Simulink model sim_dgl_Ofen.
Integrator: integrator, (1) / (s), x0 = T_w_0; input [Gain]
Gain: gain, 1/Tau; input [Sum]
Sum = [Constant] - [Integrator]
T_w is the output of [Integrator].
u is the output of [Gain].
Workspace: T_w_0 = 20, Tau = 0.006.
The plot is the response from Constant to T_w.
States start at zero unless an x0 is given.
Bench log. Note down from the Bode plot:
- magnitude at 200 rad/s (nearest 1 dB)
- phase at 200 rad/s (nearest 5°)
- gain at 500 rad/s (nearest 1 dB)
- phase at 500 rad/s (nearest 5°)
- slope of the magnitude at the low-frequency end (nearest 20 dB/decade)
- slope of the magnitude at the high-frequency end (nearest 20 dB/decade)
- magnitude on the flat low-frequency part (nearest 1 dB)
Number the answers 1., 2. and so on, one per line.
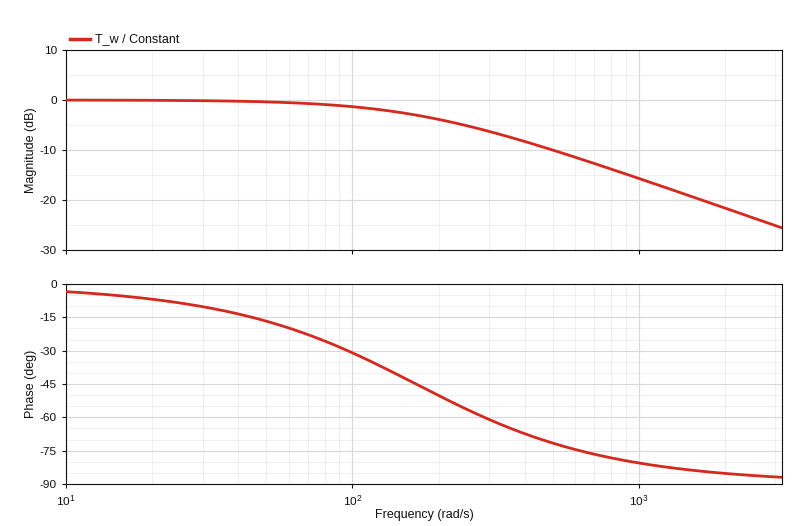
1. -4 dB
2. -50°
3. -10 dB
4. -70°
5. 0 dB/decade
6. -20 dB/decade
7. 0 dB
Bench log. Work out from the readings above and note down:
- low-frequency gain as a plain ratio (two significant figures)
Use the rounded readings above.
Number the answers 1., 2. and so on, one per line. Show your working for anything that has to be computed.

1. 10^(0 / 20) = 1.0
